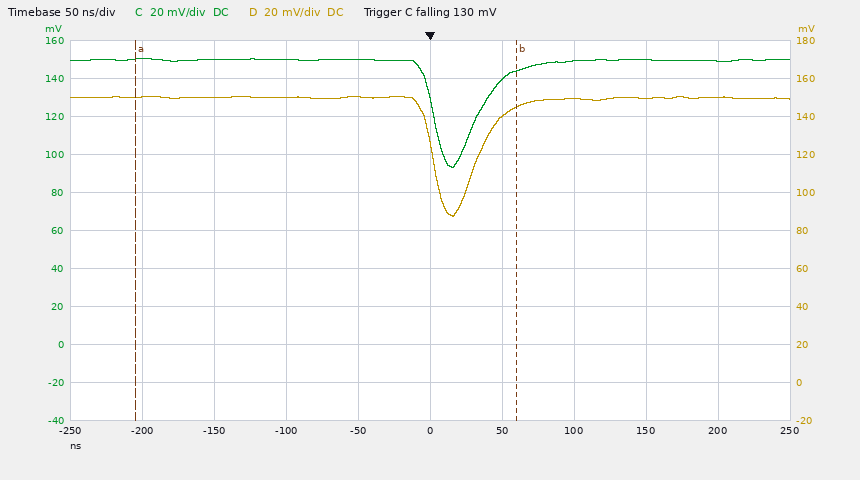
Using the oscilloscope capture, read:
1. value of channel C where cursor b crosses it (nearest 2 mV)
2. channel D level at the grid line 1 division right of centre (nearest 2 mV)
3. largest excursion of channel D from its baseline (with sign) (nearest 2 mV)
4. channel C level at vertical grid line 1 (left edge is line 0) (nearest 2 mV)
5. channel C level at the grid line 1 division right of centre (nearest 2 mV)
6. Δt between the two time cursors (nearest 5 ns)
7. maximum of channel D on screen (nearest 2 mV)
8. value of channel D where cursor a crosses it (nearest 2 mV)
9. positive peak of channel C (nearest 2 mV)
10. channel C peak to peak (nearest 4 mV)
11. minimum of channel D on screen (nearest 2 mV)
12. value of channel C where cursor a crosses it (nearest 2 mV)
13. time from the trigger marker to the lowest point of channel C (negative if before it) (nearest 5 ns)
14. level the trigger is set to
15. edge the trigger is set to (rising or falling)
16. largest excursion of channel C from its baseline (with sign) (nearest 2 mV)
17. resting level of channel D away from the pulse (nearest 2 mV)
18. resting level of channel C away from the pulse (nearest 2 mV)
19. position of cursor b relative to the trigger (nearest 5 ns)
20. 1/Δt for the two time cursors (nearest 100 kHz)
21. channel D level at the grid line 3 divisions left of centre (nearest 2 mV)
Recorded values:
144 mV
140 mV
-62 mV
150 mV
140 mV
265 ns
150 mV
150 mV
150 mV
56 mV
88 mV
150 mV
+15 ns
130 mV
falling
-56 mV
150 mV
150 mV
+60 ns
3.8 MHz
150 mV
